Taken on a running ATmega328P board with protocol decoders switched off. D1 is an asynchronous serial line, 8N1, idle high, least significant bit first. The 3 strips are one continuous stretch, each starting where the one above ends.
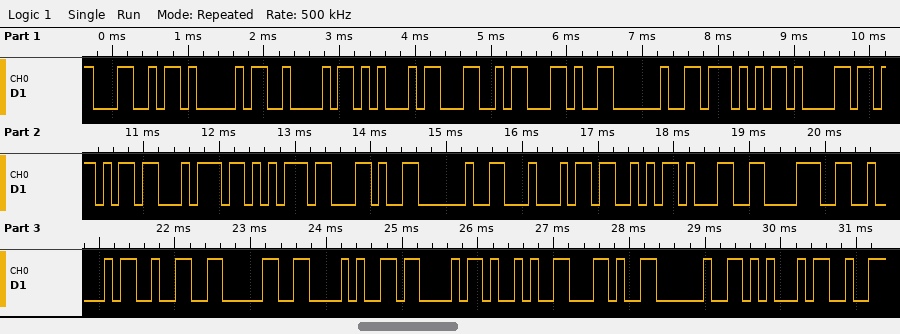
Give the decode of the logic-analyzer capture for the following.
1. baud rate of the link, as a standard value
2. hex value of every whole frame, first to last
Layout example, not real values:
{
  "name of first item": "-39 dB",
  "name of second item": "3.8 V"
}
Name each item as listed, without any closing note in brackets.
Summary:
{
  "baud rate of the link, as a standard value": "9600 baud",
  "hex value of every whole frame, first to last": "4C 41 42 45 4C 2C 20 57 61 6B 74 75 2C 20 44 53 31 38 42 32 30 28 43 29 2C 20 45"
}
